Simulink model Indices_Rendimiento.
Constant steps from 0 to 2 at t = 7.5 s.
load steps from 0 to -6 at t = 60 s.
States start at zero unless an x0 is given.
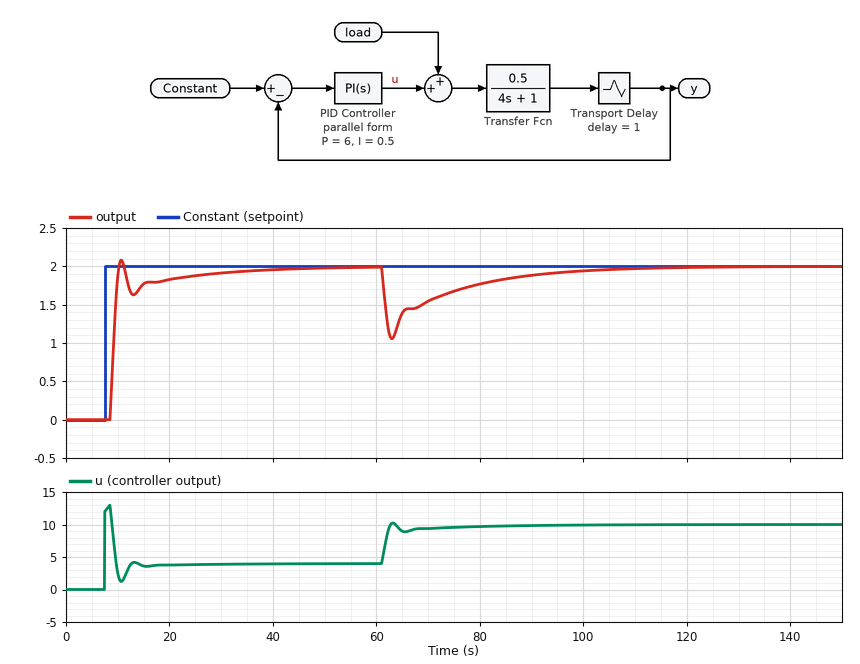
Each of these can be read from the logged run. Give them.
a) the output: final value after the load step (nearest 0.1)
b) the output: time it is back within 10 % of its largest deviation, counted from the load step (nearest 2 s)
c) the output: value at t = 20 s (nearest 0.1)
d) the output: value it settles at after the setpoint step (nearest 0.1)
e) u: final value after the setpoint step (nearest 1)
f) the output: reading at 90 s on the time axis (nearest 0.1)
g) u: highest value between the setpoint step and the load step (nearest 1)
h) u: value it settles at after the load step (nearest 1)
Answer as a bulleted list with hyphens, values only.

- 2.0
- 34 s
- 1.8
- 2.0
- 4
- 1.9
- 13
- 10
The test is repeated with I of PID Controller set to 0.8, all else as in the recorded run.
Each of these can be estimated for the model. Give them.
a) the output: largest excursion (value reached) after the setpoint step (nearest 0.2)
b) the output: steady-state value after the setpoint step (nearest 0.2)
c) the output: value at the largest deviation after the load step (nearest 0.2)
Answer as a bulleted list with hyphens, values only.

- 2.2
- 2.0
- 1.0
